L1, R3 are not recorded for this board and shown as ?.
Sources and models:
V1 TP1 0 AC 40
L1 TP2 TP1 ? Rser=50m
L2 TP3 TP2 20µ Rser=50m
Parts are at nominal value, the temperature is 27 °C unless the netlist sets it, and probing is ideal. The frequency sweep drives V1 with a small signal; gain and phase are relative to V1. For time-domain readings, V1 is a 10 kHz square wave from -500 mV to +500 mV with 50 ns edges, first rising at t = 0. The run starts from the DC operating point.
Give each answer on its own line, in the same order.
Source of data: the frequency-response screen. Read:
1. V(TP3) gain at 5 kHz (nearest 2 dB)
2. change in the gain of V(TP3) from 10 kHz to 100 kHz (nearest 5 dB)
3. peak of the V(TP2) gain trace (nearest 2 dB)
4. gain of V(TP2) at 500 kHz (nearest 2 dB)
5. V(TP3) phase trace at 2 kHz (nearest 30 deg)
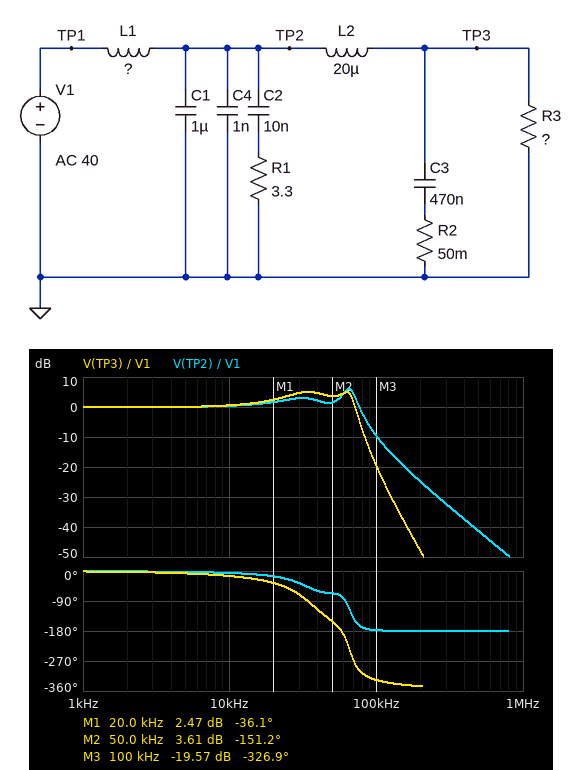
0 dB
-20 dB
6 dB
-42 dB
0 deg
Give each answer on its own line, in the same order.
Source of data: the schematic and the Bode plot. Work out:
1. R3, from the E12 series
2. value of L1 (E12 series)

8.2 Ω
12 µH
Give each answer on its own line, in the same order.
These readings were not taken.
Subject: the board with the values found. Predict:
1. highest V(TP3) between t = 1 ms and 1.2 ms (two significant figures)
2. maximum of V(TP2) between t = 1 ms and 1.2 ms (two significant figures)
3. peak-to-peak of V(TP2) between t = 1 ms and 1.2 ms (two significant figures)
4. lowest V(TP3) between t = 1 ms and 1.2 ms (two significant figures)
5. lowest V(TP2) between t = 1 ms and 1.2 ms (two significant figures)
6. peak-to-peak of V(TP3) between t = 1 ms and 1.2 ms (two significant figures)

1.1 V
900 mV
1.8 V
-1.1 V
-900 mV
2.1 V
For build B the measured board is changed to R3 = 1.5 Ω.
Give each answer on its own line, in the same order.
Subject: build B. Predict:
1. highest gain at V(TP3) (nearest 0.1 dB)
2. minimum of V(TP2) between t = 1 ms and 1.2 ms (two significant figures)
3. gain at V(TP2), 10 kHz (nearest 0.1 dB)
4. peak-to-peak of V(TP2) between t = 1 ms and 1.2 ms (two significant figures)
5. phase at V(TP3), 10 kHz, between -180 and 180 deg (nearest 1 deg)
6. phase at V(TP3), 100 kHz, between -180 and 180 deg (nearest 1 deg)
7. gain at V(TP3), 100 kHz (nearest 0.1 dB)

3.4 dB
-700 mV
-1.9 dB
1.4 V
-54 deg
74 deg
-29.0 dB
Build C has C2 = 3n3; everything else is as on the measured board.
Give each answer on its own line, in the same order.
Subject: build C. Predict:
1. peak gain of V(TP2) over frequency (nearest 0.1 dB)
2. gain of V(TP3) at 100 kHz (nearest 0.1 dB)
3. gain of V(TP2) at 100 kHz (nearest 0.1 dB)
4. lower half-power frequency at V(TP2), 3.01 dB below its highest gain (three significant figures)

6.1 dB
-19.5 dB
-9.5 dB
56.5 kHz
